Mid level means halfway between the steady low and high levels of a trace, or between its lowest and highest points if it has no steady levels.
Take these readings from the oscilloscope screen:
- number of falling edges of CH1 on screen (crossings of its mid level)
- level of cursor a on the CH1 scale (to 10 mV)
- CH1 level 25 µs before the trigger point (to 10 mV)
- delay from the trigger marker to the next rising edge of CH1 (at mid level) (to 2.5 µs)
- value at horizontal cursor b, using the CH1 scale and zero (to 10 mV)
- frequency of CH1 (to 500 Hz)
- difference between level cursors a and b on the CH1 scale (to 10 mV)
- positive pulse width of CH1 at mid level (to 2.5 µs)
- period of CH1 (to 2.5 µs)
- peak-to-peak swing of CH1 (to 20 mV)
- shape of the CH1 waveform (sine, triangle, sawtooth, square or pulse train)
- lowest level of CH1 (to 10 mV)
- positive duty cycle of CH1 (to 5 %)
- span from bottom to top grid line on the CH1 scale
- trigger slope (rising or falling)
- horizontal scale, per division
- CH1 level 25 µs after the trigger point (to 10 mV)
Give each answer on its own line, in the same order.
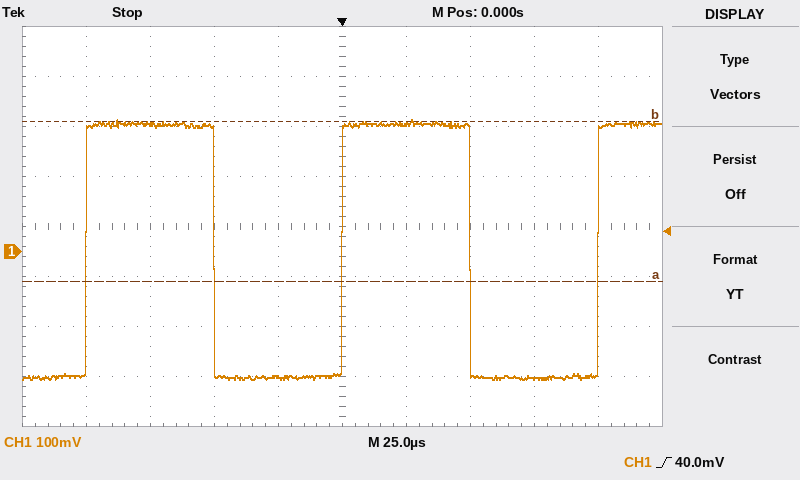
2
-60 mV
-250 mV
100.0 µs
260 mV
10.0 kHz
320 mV
50.0 µs
100.0 µs
520 mV
square
-260 mV
50 %
800 mV
rising
25 µs
260 mV
